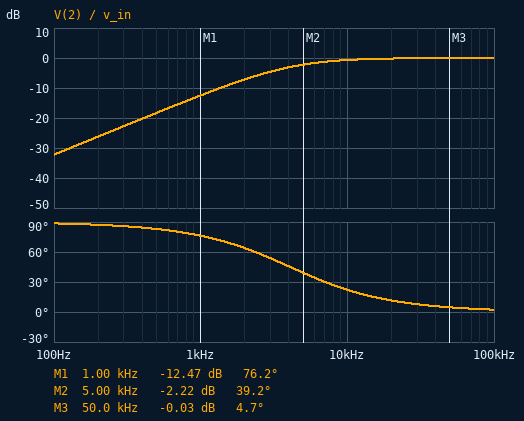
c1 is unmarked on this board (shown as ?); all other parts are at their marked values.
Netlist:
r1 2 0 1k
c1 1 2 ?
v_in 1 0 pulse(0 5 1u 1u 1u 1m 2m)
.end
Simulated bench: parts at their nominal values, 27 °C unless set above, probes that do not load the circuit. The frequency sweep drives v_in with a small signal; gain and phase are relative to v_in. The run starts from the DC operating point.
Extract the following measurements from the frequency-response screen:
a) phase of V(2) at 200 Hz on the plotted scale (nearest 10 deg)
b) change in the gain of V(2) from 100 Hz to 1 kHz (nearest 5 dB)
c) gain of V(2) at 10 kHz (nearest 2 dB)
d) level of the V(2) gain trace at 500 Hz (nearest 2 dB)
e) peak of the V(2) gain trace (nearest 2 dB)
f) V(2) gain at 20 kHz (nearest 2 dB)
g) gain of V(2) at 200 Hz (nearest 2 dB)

90 deg
20 dB
0 dB
-18 dB
0 dB
0 dB
-26 dB
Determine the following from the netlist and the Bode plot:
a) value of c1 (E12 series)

39 nF
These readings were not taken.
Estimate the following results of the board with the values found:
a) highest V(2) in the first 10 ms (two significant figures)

4.9 V
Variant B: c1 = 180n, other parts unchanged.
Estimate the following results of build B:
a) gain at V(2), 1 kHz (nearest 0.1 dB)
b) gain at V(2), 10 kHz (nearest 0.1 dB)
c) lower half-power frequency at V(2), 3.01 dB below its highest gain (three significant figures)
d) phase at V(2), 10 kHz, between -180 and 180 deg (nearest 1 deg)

-2.5 dB
0 dB
884 Hz
5 deg
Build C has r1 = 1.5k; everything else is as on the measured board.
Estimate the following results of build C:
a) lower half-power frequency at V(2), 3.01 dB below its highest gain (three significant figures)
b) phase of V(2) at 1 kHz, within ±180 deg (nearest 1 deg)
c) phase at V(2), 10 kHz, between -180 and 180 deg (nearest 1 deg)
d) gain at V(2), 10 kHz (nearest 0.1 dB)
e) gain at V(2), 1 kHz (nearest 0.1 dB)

2.72 kHz
70 deg
15 deg
-0.3 dB
-9.2 dB
